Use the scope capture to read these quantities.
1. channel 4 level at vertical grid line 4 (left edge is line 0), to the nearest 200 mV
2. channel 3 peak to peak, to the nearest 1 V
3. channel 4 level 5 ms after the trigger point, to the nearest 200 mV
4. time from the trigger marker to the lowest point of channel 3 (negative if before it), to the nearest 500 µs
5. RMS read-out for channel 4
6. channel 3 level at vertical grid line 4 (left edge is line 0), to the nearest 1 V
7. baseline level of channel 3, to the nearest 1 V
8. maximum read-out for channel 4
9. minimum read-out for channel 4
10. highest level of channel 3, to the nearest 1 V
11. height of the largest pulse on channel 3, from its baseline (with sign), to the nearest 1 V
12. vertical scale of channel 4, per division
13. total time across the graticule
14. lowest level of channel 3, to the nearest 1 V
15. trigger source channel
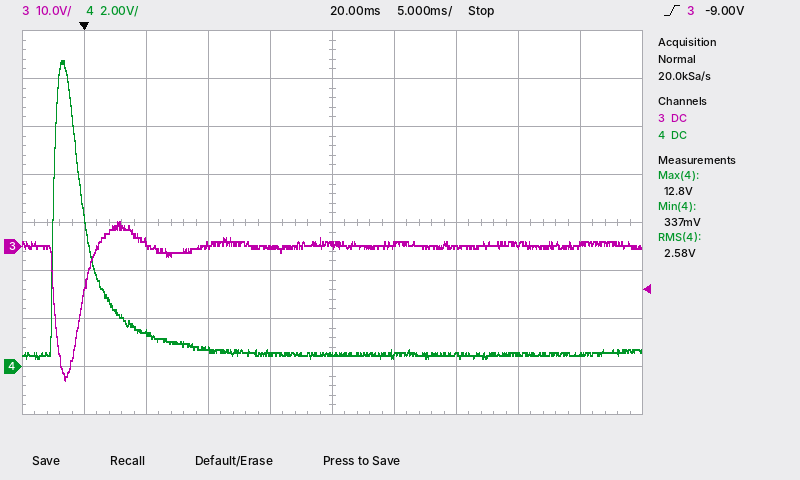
600 mV
33 V
1.4 V
-1.5 ms
2.58 V
0 V
0 V
12.8 V
337 mV
5 V
-28 V
2 V
50 ms
-28 V
channel 3
